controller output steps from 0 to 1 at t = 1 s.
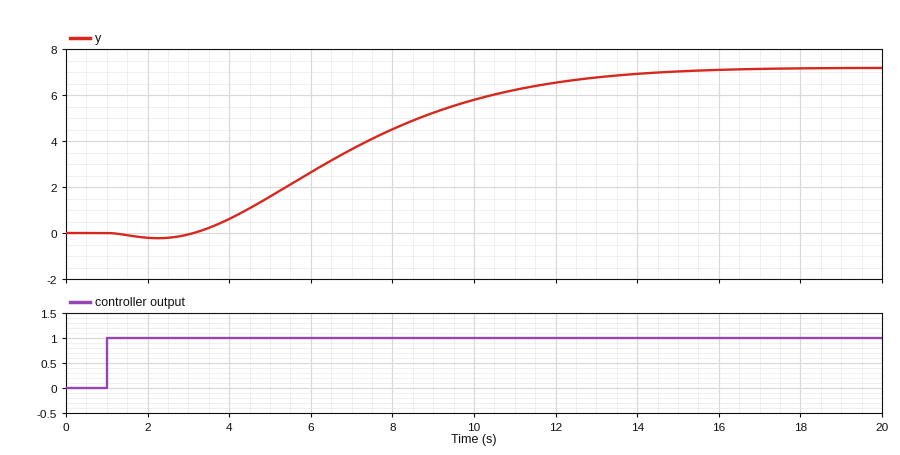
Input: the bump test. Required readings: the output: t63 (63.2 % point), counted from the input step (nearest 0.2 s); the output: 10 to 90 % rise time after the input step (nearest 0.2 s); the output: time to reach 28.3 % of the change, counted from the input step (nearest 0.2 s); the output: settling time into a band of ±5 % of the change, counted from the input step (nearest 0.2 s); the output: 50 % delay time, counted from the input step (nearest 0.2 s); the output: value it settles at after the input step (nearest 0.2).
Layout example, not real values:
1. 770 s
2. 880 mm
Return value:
1. 7.0 s
2. 7.6 s
3. 4.4 s
4. 12.2 s
5. 6.0 s
6. 7.2
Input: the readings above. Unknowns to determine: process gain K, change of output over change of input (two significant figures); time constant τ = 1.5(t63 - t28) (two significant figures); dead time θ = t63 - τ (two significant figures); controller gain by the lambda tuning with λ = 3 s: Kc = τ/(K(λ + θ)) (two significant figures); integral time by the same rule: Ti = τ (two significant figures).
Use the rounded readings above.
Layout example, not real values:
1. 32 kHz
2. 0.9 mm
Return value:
1. 7.2
2. 3.9 s
3. 3.1 s
4. 0.089
5. 3.9 s
